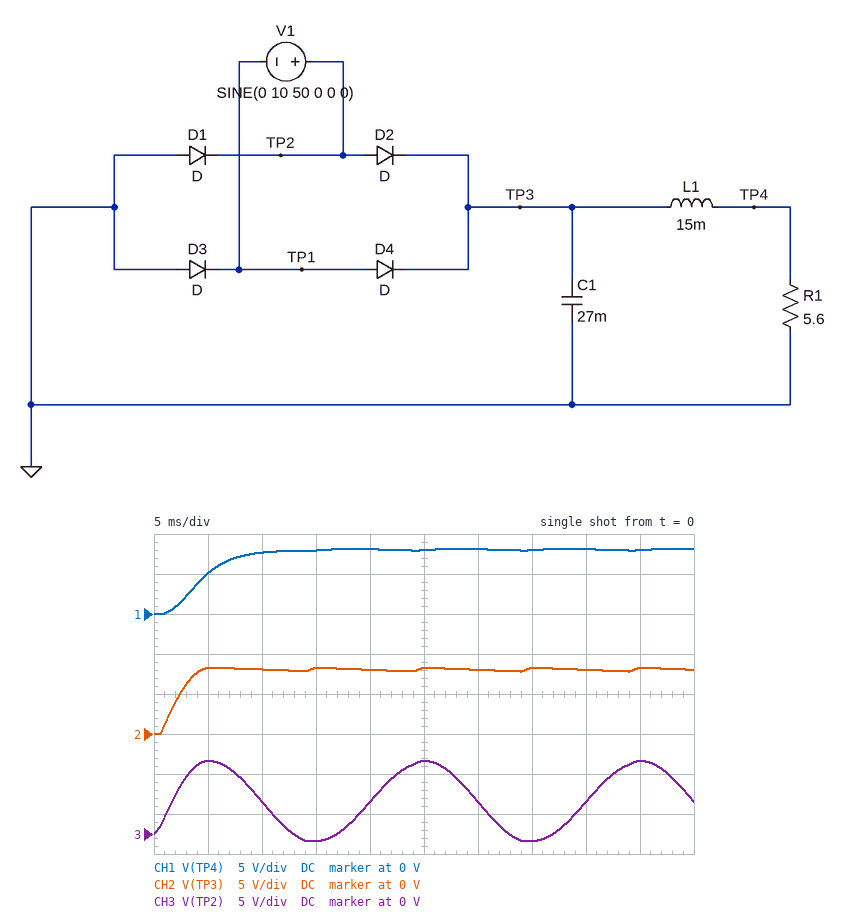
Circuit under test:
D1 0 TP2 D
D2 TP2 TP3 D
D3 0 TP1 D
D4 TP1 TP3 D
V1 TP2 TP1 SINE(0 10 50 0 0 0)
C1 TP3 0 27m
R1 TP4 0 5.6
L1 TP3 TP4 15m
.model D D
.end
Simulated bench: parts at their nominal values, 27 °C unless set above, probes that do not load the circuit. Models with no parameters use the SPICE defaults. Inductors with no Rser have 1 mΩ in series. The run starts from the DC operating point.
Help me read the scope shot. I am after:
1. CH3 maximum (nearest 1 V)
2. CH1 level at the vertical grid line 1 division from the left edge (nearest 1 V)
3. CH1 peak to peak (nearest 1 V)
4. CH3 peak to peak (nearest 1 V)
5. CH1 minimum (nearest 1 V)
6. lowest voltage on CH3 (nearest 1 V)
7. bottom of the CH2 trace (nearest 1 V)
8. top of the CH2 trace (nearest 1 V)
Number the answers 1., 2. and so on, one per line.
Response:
1. 9 V
2. 5 V
3. 8 V
4. 10 V
5. 0 V
6. -1 V
7. 0 V
8. 8 V
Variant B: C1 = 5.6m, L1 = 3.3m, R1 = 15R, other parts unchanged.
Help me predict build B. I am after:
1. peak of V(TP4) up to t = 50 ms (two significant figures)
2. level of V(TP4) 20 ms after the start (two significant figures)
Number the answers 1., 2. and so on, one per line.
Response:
1. 8.3 V
2. 7.9 V
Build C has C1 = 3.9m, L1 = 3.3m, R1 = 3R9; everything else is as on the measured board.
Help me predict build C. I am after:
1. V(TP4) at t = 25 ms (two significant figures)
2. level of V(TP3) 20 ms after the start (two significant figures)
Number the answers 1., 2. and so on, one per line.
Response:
1. 7.7 V
2. 6.1 V
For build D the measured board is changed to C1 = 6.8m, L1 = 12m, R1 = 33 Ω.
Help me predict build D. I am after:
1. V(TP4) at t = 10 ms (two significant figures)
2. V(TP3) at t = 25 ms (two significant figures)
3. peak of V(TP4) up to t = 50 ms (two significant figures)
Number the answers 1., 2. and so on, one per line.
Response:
1. 8.2 V
2. 8.3 V
3. 8.3 V
